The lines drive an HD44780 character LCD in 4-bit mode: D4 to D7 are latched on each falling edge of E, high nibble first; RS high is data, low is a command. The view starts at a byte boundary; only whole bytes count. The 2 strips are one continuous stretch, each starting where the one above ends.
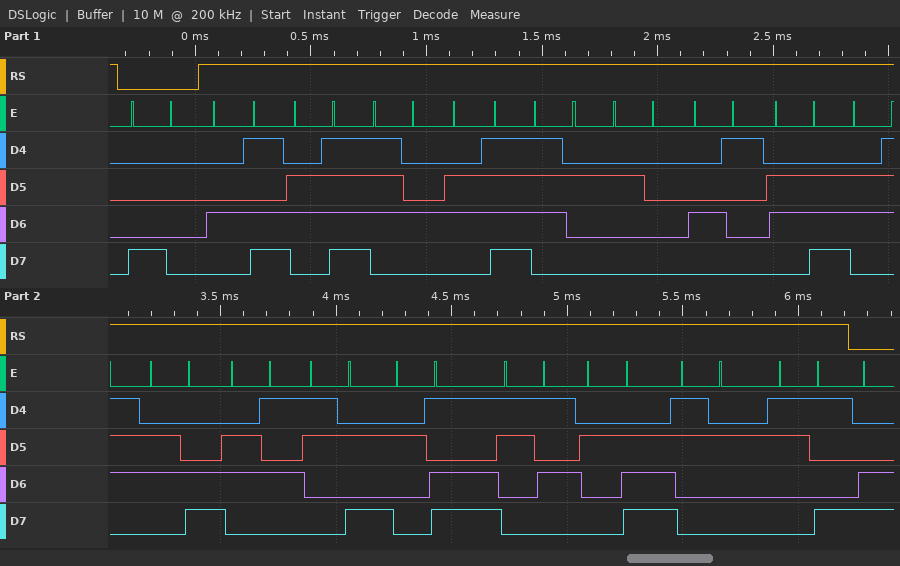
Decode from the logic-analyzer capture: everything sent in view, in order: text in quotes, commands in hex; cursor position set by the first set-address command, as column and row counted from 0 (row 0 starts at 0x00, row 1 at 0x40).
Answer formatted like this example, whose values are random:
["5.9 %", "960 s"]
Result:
["0x80 \"Motor Angle:-5.29\"", "column 0, row 0"]
